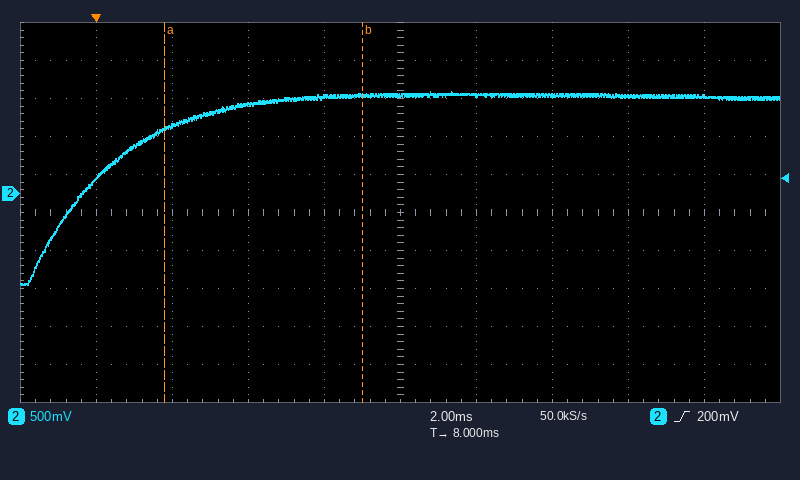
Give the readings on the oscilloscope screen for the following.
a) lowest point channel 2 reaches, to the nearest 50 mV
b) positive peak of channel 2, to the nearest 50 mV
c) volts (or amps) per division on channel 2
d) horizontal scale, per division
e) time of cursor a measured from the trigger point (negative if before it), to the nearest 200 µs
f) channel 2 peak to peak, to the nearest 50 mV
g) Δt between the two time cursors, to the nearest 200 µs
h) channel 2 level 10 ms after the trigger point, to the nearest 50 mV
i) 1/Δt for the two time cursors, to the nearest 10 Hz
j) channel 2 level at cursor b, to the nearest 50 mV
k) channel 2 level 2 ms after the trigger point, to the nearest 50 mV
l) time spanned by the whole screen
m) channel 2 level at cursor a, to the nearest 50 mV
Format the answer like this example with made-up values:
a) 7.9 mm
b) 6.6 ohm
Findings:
a) -1.20 V
b) 1.35 V
c) 500 mV
d) 2 ms
e) +1.8 ms
f) 2.55 V
g) 5.2 ms
h) 1.30 V
i) 190 Hz
j) 1.30 V
k) 900 mV
l) 20 ms
m) 850 mV
